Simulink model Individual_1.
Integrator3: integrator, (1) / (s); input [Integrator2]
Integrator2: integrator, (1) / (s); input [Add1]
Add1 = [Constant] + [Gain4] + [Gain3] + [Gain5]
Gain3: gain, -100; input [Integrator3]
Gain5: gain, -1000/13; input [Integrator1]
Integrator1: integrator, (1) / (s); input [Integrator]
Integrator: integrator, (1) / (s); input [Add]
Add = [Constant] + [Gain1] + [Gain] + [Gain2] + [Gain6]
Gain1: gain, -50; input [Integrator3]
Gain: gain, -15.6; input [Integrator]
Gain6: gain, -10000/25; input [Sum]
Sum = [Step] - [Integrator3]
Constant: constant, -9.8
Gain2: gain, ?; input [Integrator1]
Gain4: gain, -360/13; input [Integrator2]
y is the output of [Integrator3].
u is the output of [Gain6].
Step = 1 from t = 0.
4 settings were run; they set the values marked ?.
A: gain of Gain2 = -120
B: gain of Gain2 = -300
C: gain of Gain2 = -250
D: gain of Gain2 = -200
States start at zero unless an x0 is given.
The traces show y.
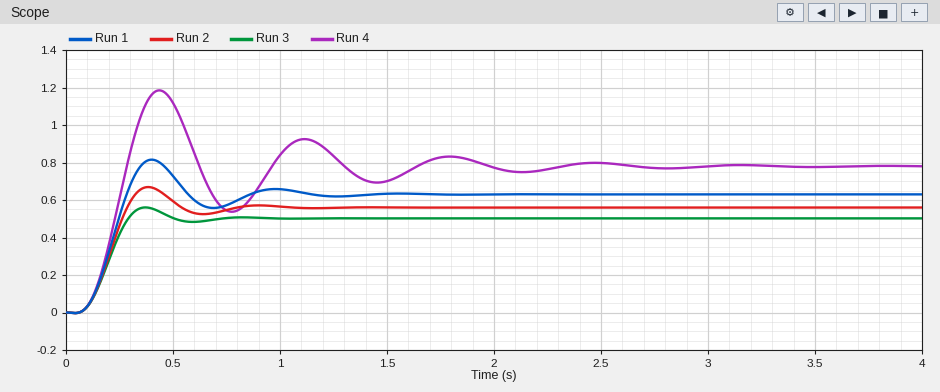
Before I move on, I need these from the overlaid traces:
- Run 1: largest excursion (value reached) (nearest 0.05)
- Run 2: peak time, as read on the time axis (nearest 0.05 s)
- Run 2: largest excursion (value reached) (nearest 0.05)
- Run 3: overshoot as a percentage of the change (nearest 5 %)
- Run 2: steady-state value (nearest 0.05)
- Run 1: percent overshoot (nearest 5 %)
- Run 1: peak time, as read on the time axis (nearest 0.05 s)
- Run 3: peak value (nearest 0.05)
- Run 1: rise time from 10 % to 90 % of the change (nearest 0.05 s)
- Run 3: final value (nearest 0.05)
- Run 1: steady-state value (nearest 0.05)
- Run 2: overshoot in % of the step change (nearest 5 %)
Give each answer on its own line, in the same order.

0.80
0.40 s
0.65
10 %
0.55
30 %
0.40 s
0.55
0.15 s
0.50
0.65
20 %
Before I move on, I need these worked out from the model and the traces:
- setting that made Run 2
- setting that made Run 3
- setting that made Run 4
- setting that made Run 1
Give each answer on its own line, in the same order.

C
B
A
D
